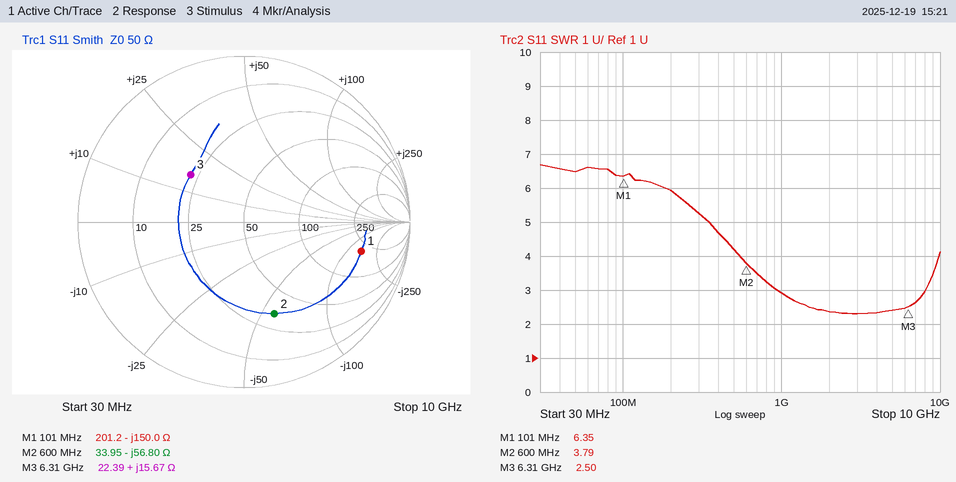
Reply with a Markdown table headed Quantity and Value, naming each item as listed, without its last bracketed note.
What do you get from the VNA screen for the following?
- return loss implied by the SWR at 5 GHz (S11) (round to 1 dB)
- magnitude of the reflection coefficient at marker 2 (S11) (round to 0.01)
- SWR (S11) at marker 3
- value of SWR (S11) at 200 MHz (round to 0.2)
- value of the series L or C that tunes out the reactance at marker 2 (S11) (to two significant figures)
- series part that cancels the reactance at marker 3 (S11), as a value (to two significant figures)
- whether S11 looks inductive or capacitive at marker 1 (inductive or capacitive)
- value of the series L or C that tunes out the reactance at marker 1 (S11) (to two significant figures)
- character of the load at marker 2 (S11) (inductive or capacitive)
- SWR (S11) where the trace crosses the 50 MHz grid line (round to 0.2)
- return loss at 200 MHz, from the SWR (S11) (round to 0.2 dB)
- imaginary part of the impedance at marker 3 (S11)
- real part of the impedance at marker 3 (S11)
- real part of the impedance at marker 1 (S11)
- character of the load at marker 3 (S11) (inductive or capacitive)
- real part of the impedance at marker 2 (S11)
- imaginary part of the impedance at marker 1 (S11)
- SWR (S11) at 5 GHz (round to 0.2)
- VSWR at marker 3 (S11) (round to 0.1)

| Quantity | Value |
|---|---|
| return loss implied by the SWR at 5 GHz (S11) | 8 dB |
| magnitude of the reflection coefficient at marker 2 (S11) | 0.58 |
| SWR (S11) at marker 3 | 2.50 |
| value of SWR (S11) at 200 MHz | 6.0 |
| value of the series L or C that tunes out the reactance at marker 2 (S11) | 15 nH |
| series part that cancels the reactance at marker 3 (S11), as a value | 1.6 pF |
| whether S11 looks inductive or capacitive at marker 1 | capacitive |
| value of the series L or C that tunes out the reactance at marker 1 (S11) | 240 nH |
| character of the load at marker 2 (S11) | capacitive |
| SWR (S11) where the trace crosses the 50 MHz grid line | 6.4 |
| return loss at 200 MHz, from the SWR (S11) | 3.0 dB |
| imaginary part of the impedance at marker 3 | +15.67 Ω |
| real part of the impedance at marker 3 | 22.39 Ω |
| real part of the impedance at marker 1 | 201.2 Ω |
| character of the load at marker 3 (S11) | inductive |
| real part of the impedance at marker 2 | 33.95 Ω |
| imaginary part of the impedance at marker 1 | -150.0 Ω |
| SWR (S11) at 5 GHz | 2.4 |
| VSWR at marker 3 (S11) | 2.5 |
